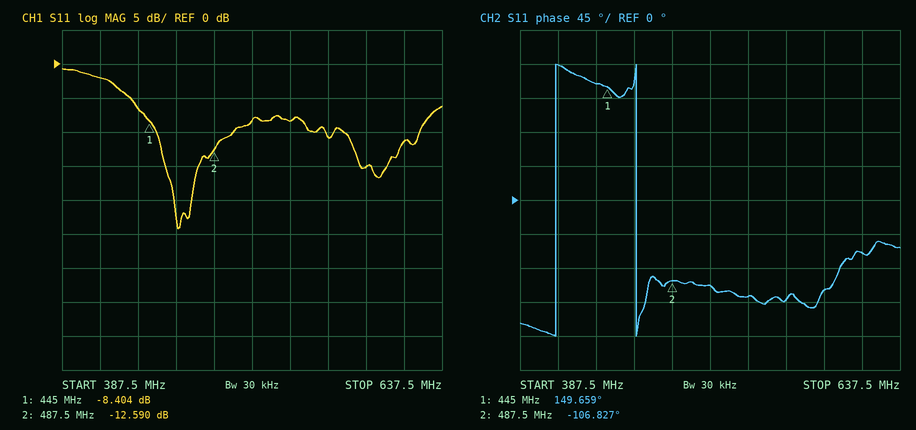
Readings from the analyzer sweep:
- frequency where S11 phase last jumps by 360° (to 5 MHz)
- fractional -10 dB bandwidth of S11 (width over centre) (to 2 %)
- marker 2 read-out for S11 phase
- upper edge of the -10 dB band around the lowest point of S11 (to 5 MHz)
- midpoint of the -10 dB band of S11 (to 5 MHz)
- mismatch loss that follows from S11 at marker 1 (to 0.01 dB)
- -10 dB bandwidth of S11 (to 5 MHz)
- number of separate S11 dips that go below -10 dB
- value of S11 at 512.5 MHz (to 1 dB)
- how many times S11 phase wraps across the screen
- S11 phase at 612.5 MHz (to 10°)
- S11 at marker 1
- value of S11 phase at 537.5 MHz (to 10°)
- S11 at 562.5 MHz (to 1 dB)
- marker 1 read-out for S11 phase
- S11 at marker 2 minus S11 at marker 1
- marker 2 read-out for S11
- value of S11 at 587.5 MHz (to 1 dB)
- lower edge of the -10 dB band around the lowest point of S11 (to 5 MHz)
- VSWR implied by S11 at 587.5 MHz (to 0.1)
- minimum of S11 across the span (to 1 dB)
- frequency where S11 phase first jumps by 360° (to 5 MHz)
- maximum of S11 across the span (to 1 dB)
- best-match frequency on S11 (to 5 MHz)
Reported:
465 MHz
10 %
-106.827°
500 MHz
475 MHz
0.68 dB
50 MHz
2
-8 dB
2
-70°
-8.404 dB
-130°
-11 dB
149.659°
-4.186 dB
-12.590 dB
-15 dB
450 MHz
1.4
-24 dB
410 MHz
-1 dB
465 MHz
